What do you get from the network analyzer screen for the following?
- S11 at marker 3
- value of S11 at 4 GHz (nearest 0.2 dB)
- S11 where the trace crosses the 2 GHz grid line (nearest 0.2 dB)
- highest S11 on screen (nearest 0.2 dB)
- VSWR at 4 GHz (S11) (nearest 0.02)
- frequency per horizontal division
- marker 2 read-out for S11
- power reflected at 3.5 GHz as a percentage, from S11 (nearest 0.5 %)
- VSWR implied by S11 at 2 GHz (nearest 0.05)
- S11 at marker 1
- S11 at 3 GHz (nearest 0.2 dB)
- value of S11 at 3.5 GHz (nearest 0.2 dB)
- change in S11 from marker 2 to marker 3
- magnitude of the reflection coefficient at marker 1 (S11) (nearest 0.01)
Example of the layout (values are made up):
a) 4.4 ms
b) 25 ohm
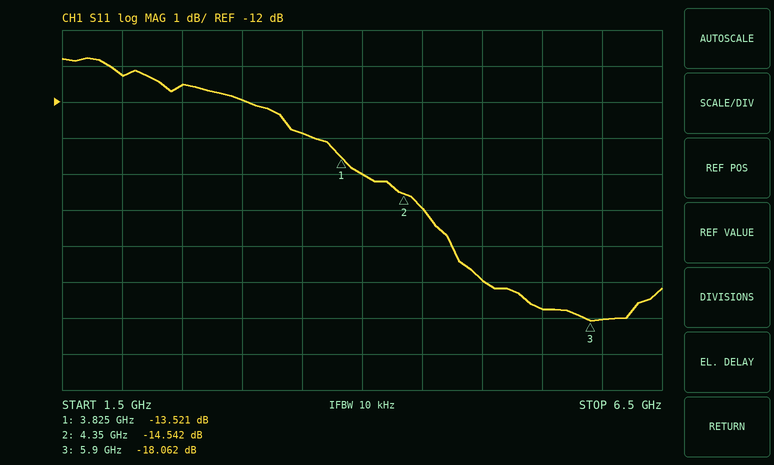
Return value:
a) -18.062 dB
b) -14.0 dB
c) -11.2 dB
d) -10.8 dB
e) 1.50
f) 500 MHz
g) -14.542 dB
h) 5.0 %
i) 1.75
j) -13.521 dB
k) -12.0 dB
l) -12.8 dB
m) -3.520 dB
n) 0.21
